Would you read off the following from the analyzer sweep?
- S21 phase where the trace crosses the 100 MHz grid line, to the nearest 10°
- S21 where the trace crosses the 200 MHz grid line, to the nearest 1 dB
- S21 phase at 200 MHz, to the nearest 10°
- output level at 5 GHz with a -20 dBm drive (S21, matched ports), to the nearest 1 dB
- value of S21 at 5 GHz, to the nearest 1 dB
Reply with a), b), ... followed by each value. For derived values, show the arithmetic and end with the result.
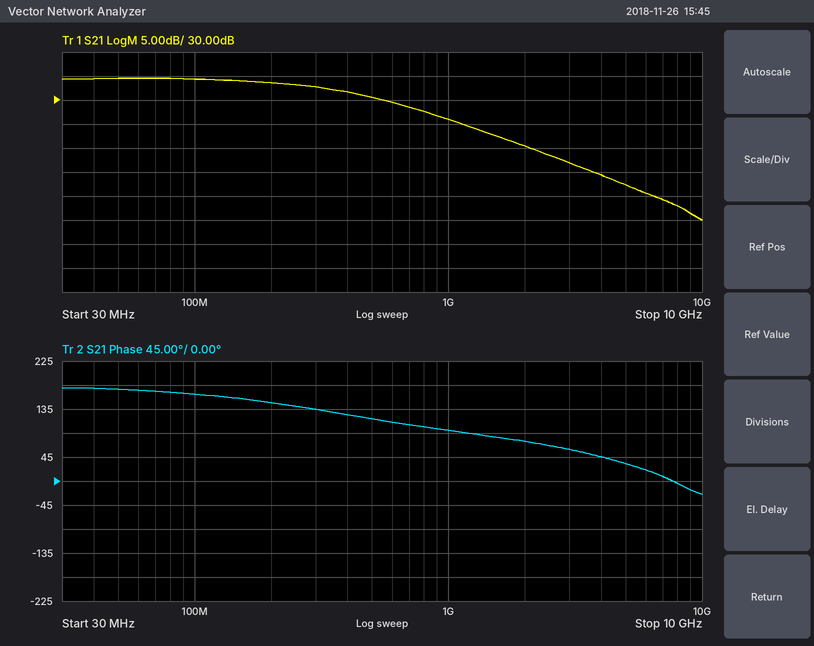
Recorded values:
a) 160°
b) 34 dB
c) 150°
d) -20 dBm + (12 dB) = -8 dBm
e) 12 dB
